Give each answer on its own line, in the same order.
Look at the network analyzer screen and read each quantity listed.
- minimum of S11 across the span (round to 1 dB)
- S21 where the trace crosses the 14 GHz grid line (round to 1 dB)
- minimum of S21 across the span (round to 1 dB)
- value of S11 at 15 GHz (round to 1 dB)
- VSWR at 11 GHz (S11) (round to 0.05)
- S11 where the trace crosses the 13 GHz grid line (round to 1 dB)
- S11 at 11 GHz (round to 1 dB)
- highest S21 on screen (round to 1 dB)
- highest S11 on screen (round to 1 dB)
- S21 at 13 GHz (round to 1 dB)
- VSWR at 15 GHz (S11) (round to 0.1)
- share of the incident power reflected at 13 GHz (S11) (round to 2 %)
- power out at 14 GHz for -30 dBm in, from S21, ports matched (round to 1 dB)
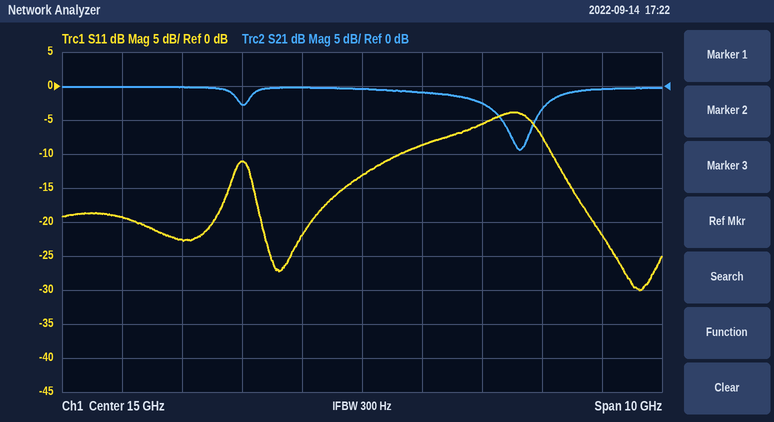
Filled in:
-30 dB
0 dB
-9 dB
-13 dB
1.25
-11 dB
-19 dB
0 dB
-4 dB
-3 dB
1.6
8 %
-30 dBm
